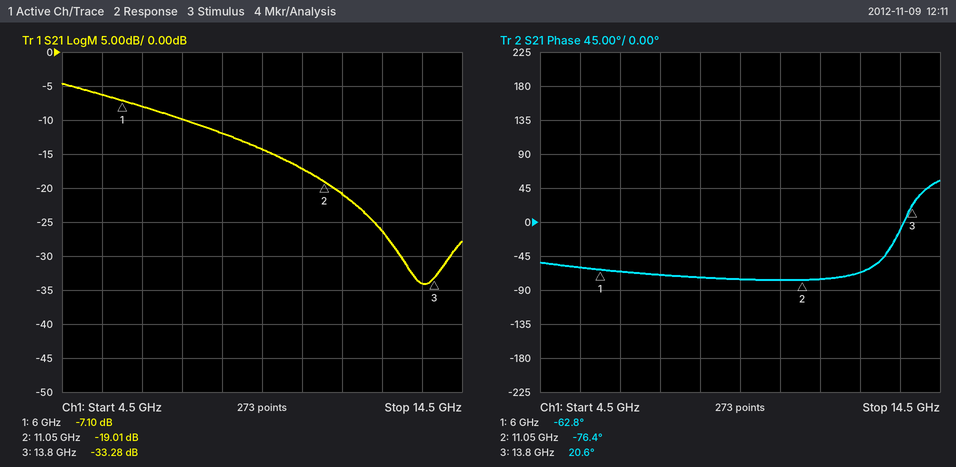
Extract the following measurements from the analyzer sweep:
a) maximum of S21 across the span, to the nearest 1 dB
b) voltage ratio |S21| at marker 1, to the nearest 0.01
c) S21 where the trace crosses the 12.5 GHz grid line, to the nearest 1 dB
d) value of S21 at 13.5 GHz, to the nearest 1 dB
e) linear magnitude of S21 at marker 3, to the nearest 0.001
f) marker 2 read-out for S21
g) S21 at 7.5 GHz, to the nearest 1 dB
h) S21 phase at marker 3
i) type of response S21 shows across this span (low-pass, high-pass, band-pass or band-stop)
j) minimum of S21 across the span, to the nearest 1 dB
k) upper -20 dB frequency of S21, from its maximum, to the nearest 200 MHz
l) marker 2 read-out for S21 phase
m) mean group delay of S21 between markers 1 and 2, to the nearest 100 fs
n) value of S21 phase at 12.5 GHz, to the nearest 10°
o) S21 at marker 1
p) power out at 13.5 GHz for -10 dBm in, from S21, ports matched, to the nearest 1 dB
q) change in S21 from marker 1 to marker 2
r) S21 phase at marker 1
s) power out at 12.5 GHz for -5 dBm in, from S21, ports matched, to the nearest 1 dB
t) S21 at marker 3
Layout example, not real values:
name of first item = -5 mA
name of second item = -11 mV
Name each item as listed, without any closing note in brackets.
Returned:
maximum of S21 across the span, to the nearest 1 dB = -5 dB
voltage ratio |S21| at marker 1, to the nearest 0.01 = 0.44
S21 where the trace crosses the 12.5 GHz grid line, to the nearest 1 dB = -26 dB
value of S21 at 13.5 GHz, to the nearest 1 dB = -34 dB
linear magnitude of S21 at marker 3, to the nearest 0.001 = 0.022
marker 2 read-out for S21 = -19.01 dB
S21 at 7.5 GHz, to the nearest 1 dB = -10 dB
S21 phase at marker 3 = 20.6°
type of response S21 shows across this span = low-pass
minimum of S21 across the span, to the nearest 1 dB = -34 dB
upper -20 dB frequency of S21, from its maximum, to the nearest 200 MHz = 12.2 GHz
marker 2 read-out for S21 phase = -76.4°
mean group delay of S21 between markers 1 and 2, to the nearest 100 fs = 7.5 ps
value of S21 phase at 12.5 GHz, to the nearest 10° = -70°
S21 at marker 1 = -7.10 dB
power out at 13.5 GHz for -10 dBm in, from S21, ports matched, to the nearest 1 dB = -44 dBm
change in S21 from marker 1 to marker 2 = -11.91 dB
S21 phase at marker 1 = -62.8°
power out at 12.5 GHz for -5 dBm in, from S21, ports matched, to the nearest 1 dB = -31 dBm
S21 at marker 3 = -33.28 dB
